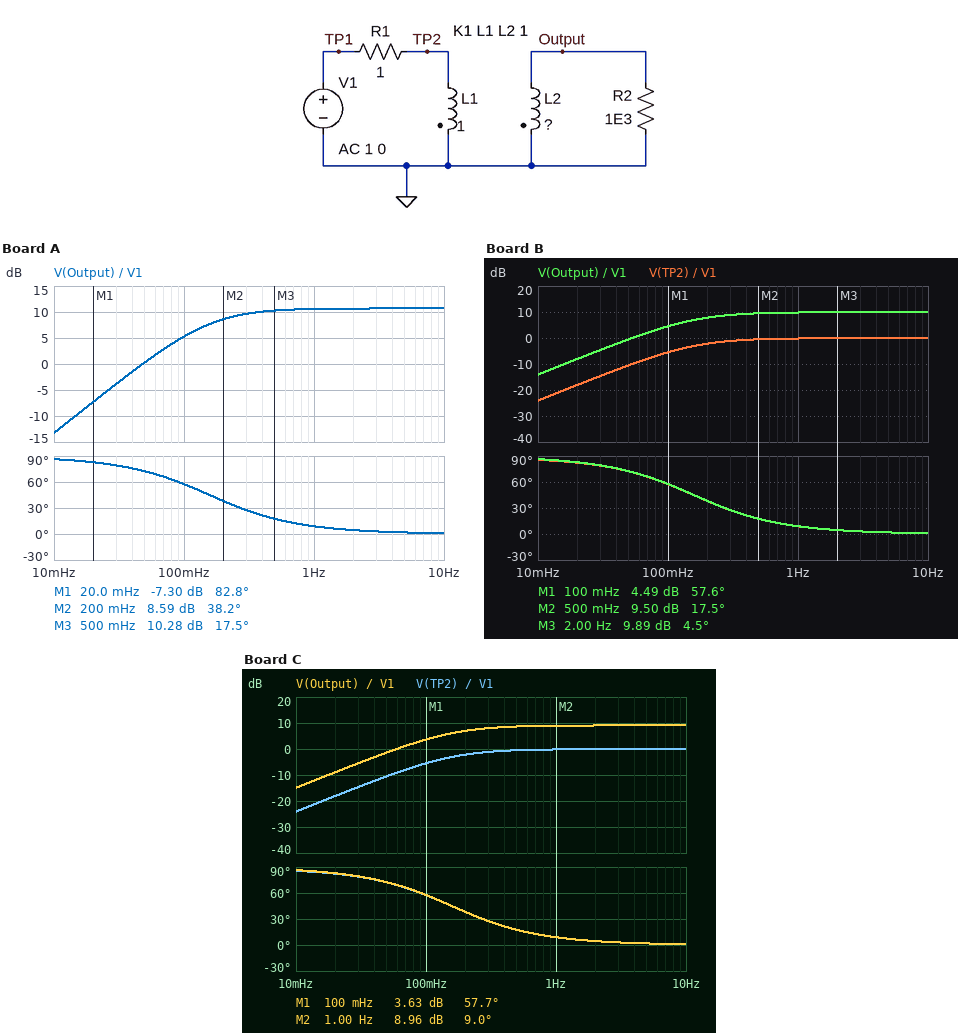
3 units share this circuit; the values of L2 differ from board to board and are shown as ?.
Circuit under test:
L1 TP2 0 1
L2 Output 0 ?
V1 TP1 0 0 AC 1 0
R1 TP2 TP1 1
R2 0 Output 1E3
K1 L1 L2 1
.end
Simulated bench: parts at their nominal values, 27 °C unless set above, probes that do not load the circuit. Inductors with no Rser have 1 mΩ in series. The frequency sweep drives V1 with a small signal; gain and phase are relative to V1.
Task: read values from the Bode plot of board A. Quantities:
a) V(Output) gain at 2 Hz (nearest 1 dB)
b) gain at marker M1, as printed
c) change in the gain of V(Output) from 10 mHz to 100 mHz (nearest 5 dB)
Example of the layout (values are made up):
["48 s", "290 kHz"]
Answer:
["11 dB", "-7.30 dB", "20 dB"]
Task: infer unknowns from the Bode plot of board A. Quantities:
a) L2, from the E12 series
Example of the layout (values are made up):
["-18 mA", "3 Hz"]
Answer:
["12 H"]
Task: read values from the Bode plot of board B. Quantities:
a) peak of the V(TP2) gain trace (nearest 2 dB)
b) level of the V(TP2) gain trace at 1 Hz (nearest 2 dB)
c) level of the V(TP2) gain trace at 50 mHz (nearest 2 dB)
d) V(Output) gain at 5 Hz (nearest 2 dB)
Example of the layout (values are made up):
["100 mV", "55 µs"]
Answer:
["0 dB", "0 dB", "-10 dB", "10 dB"]
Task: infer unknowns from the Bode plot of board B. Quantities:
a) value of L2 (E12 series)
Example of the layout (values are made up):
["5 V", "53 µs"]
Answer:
["10 H"]
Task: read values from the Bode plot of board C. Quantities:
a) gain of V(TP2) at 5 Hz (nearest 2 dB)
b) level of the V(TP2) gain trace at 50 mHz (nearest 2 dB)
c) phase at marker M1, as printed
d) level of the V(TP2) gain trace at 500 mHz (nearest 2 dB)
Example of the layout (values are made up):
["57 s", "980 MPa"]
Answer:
["0 dB", "-10 dB", "57.7 deg", "0 dB"]
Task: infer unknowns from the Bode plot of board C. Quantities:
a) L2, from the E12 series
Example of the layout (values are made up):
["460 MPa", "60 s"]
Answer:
["8.2 H"]
